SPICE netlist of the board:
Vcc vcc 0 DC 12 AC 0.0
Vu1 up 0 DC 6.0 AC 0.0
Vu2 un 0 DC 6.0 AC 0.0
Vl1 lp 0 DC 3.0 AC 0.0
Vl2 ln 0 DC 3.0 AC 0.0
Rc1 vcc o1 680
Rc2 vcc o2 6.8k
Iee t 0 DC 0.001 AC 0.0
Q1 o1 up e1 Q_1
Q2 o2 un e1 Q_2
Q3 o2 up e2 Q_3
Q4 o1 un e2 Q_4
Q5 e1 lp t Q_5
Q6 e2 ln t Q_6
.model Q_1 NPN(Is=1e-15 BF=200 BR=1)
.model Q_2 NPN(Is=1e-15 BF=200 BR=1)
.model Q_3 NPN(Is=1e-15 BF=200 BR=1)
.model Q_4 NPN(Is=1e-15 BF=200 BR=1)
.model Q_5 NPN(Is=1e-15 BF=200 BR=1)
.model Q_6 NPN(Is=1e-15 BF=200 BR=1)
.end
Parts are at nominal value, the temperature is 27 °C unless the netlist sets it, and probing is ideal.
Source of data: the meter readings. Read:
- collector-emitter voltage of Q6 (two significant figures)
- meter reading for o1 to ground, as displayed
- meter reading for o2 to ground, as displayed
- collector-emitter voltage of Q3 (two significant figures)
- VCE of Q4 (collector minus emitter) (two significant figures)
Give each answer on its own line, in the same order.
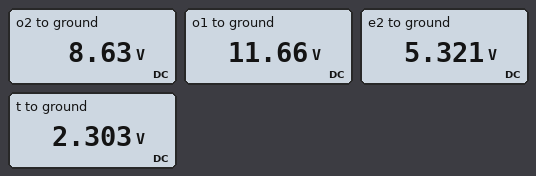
3.0 V
11.66 V
8.63 V
3.3 V
6.3 V
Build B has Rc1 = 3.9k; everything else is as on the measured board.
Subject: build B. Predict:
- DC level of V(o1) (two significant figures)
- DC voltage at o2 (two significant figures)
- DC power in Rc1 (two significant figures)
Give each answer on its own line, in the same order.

10 V
8.6 V
960 µW
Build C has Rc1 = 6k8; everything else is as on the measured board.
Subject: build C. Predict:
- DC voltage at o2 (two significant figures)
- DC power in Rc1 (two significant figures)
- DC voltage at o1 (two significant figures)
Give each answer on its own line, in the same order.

8.6 V
1.7 mW
8.6 V
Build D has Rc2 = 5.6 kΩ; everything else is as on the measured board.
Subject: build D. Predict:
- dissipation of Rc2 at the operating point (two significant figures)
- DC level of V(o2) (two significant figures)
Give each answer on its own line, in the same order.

1.4 mW
9.2 V
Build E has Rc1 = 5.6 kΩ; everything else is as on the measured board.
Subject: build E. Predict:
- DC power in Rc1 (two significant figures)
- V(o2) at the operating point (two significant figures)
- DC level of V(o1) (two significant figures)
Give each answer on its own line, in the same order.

1.4 mW
8.6 V
9.2 V
